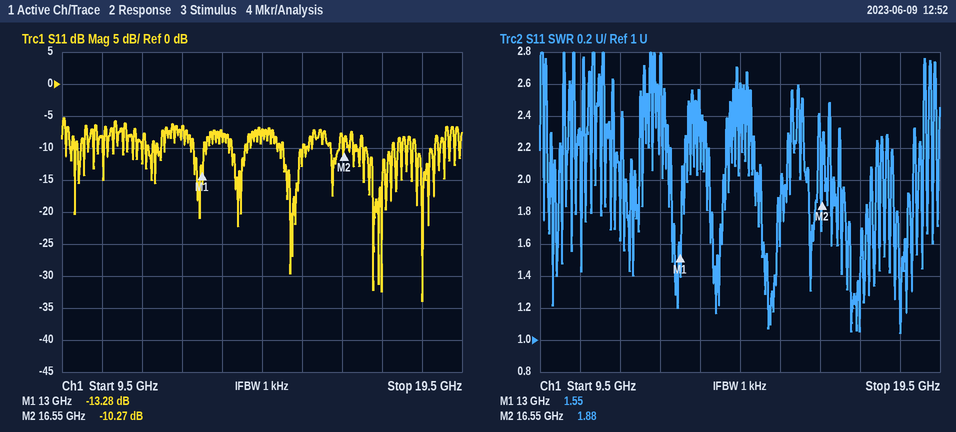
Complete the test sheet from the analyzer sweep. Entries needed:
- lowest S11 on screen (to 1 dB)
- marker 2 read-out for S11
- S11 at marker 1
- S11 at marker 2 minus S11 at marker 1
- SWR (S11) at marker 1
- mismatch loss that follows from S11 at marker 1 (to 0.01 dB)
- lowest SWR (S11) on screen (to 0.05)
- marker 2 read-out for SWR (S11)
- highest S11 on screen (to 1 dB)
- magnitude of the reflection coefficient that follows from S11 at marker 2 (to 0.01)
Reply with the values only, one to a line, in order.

-34 dB
-10.27 dB
-13.28 dB
3.01 dB
1.55
0.21 dB
1.05
1.88
-5 dB
0.31
